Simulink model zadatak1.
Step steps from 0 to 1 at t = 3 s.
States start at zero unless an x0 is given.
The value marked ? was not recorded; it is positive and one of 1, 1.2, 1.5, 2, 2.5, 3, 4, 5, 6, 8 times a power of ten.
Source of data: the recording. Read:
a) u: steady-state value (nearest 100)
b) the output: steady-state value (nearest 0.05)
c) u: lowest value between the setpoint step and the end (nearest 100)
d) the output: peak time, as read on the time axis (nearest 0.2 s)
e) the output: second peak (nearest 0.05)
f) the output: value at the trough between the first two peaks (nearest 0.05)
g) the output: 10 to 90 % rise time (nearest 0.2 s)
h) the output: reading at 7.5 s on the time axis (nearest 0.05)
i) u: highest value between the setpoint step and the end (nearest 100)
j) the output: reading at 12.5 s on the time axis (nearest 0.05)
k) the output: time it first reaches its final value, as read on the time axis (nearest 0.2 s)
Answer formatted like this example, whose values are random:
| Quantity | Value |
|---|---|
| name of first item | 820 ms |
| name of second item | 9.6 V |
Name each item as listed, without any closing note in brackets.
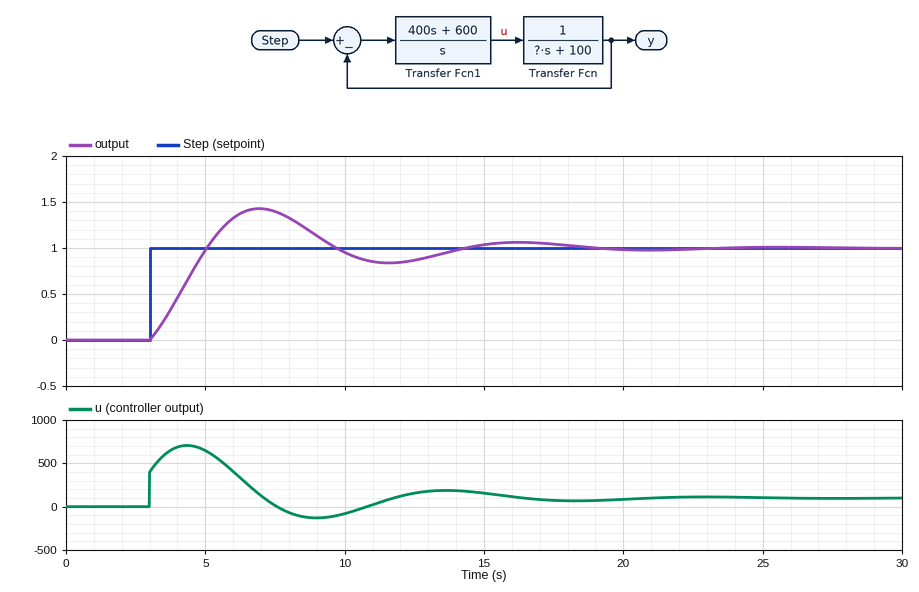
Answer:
| Quantity | Value |
|---|---|
| u: steady-state value | 100 |
| the output: steady-state value | 1.00 |
| u: lowest value between the setpoint step and the end | -100 |
| the output: peak time, as read on the time axis | 7.0 s |
| the output: second peak | 1.05 |
| the output: value at the trough between the first two peaks | 0.85 |
| the output: 10 to 90 % rise time | 1.6 s |
| the output: reading at 7.5 s on the time axis | 1.40 |
| u: highest value between the setpoint step and the end | 700 |
| the output: reading at 12.5 s on the time axis | 0.85 |
| the output: time it first reaches its final value, as read on the time axis | 5.0 s |
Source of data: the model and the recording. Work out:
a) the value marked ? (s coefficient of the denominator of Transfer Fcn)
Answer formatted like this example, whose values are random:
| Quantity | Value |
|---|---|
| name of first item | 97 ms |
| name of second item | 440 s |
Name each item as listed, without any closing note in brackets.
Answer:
| Quantity | Value |
|---|---|
| the value marked ? | 1200 |
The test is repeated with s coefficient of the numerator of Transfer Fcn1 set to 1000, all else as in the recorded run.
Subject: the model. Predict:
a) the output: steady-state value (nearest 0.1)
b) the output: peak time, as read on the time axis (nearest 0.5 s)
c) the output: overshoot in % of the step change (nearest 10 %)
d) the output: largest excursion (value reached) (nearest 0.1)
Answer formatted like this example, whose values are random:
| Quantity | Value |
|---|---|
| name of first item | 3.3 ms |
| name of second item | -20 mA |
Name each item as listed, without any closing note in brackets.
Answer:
| Quantity | Value |
|---|---|
| the output: steady-state value | 1.0 |
| the output: peak time, as read on the time axis | 6.5 s |
| the output: overshoot in % of the step change | 20 % |
| the output: largest excursion (value reached) | 1.2 |
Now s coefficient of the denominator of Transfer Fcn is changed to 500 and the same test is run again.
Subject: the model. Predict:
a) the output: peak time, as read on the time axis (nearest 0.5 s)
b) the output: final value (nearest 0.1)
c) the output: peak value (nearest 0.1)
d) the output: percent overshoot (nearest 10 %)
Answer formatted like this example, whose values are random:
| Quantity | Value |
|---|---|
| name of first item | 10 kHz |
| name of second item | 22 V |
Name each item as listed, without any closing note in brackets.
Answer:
| Quantity | Value |
|---|---|
| the output: peak time, as read on the time axis | 5.5 s |
| the output: final value | 1.0 |
| the output: peak value | 1.3 |
| the output: percent overshoot | 30 % |
